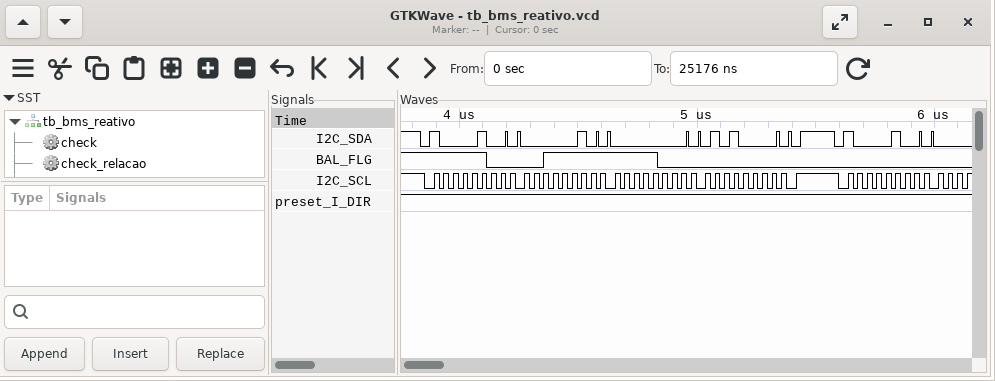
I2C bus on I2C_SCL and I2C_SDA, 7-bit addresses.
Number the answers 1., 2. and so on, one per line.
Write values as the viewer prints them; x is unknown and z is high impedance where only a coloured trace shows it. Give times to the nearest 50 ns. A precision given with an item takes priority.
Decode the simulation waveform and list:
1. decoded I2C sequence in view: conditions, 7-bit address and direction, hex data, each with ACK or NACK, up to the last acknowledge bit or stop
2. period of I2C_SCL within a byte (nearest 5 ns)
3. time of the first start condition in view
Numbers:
1. start, address 42 write ACK, 02 ACK, 00 ACK, 50 ACK, stop, start, address 42 write ACK
2. 40 ns
3. 3850 ns
